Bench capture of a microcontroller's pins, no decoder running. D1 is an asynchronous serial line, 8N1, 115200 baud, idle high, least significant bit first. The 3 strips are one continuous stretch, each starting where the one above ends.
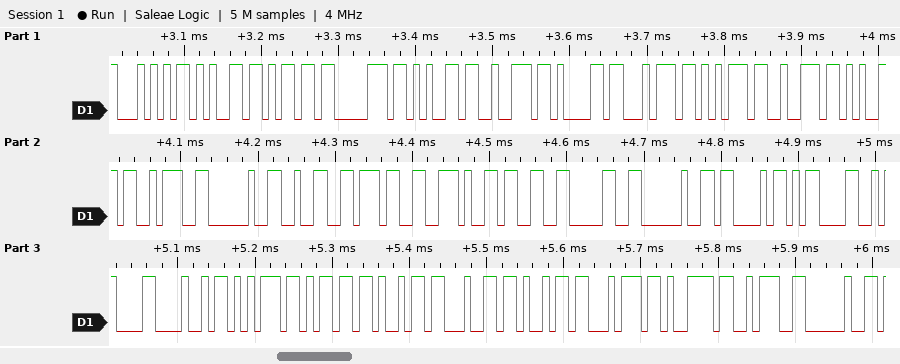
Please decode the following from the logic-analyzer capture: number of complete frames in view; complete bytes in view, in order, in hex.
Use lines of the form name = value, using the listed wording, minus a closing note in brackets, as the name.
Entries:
number of complete frames in view = 32
complete bytes in view, in order, in hex = 54 65 6D 70 65 72 61 74 75 72 65 3A 20 32 37 2E 33 30 20 43 0D 0A 48 75 6D 69 64 69 74 79 3A 20
